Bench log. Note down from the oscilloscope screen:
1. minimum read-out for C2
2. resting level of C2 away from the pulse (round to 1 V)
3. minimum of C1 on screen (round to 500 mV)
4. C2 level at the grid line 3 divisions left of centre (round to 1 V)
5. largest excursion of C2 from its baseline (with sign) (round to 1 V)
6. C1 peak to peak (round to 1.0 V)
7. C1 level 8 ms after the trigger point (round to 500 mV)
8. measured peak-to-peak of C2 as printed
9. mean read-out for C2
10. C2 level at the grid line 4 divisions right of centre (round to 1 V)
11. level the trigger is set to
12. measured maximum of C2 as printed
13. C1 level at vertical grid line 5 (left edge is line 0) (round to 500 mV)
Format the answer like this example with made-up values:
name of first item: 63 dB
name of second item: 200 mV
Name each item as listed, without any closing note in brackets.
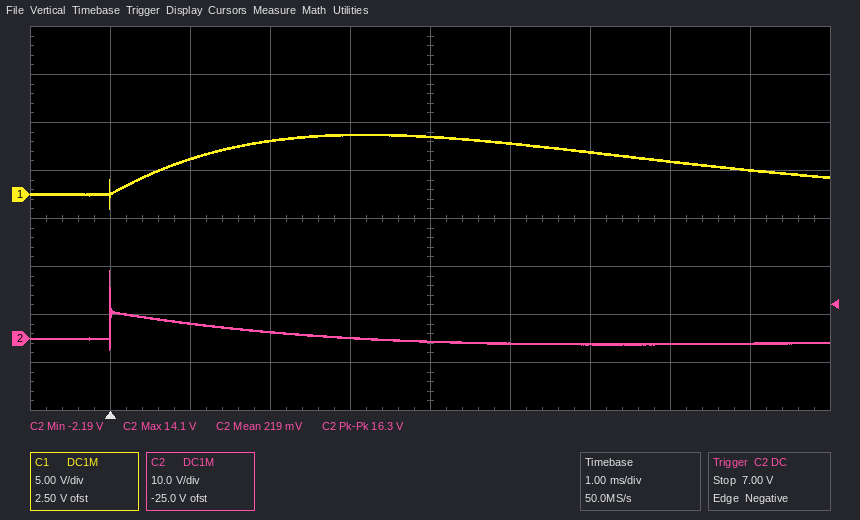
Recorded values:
minimum read-out for C2: -2.19 V
resting level of C2 away from the pulse: -1 V
minimum of C1 on screen: -1.5 V
C2 level at the grid line 3 divisions left of centre: 3 V
largest excursion of C2 from its baseline (with sign): +15 V
C1 peak to peak: 8.0 V
C1 level 8 ms after the trigger point: 2.5 V
measured peak-to-peak of C2 as printed: 16.3 V
mean read-out for C2: 219 mV
C2 level at the grid line 4 divisions right of centre: -1 V
level the trigger is set to: 7.00 V
measured maximum of C2 as printed: 14.1 V
C1 level at vertical grid line 5 (left edge is line 0): 6.0 V
